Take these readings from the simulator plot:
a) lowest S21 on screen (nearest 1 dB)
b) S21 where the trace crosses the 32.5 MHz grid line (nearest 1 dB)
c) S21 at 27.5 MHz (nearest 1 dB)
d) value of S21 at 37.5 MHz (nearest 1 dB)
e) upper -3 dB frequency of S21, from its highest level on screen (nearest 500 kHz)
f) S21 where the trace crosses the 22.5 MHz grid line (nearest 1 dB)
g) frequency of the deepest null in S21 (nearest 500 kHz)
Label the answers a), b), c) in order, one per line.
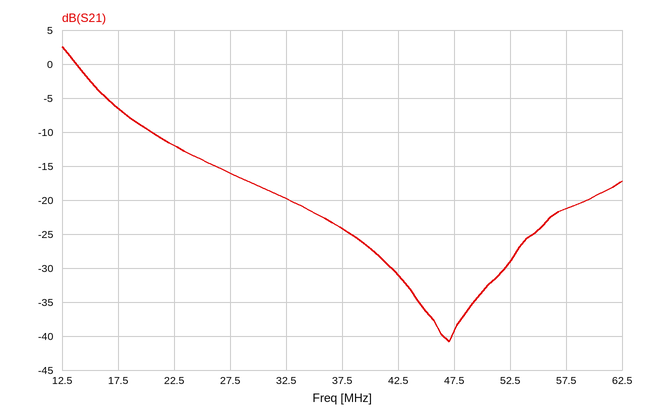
a) -41 dB
b) -20 dB
c) -16 dB
d) -24 dB
e) 14.0 MHz
f) -12 dB
g) 47.0 MHz
